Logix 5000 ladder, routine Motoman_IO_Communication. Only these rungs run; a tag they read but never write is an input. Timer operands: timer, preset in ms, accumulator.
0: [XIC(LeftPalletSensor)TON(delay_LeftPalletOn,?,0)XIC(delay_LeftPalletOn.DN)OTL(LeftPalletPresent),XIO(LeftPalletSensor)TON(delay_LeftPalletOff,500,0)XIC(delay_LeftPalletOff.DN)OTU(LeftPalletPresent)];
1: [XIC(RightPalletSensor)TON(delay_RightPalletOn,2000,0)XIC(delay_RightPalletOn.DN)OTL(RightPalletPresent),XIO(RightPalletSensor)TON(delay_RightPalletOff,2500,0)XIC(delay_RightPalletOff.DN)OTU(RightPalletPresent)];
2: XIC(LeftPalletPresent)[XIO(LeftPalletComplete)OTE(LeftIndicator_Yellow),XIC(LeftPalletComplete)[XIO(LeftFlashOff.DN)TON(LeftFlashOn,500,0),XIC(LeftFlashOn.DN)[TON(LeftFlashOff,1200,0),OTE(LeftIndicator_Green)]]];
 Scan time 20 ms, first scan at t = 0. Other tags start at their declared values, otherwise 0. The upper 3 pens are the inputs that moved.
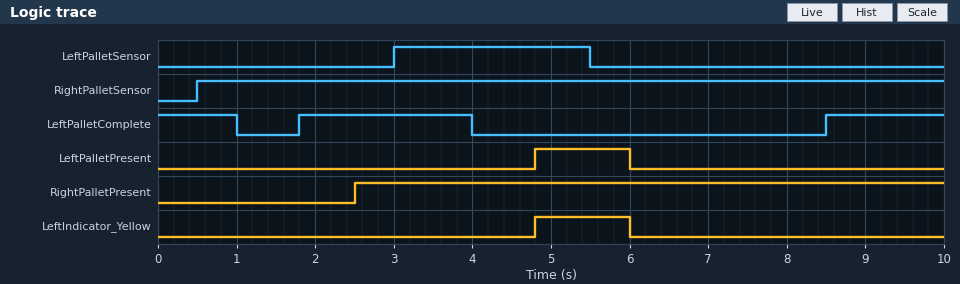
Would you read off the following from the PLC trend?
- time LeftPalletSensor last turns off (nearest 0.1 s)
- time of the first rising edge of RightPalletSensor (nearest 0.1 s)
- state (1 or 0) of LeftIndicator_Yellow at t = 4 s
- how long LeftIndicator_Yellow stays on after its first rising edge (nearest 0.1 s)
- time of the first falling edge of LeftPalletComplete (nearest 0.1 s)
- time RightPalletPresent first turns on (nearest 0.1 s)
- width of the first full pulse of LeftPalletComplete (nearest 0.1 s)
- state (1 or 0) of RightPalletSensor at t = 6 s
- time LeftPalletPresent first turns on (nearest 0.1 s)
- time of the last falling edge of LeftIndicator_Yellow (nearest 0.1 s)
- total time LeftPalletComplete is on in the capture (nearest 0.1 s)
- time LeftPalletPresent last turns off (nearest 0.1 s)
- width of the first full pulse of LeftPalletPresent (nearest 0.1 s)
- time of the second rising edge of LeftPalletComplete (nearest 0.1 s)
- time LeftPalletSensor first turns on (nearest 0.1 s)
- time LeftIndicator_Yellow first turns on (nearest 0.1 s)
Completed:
5.5 s
0.5 s
0
1.2 s
1.0 s
2.5 s
2.2 s
1
4.8 s
6.0 s
4.7 s
6.0 s
1.2 s
8.5 s
3.0 s
4.8 s
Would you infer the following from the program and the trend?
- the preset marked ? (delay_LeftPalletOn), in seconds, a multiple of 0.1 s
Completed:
1.8 s
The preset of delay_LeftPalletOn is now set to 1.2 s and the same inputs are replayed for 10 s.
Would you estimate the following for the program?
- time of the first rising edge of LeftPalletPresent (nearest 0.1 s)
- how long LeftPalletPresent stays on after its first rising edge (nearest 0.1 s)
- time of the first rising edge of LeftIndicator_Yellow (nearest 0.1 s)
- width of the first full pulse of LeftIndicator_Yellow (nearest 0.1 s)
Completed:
4.2 s
1.8 s
4.2 s
1.8 s
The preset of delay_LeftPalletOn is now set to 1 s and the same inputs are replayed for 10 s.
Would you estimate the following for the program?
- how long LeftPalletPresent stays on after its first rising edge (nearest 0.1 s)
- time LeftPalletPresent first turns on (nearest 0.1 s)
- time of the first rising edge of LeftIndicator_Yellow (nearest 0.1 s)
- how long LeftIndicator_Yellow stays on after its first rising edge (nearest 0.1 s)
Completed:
2.0 s
4.0 s
4.0 s
2.0 s
